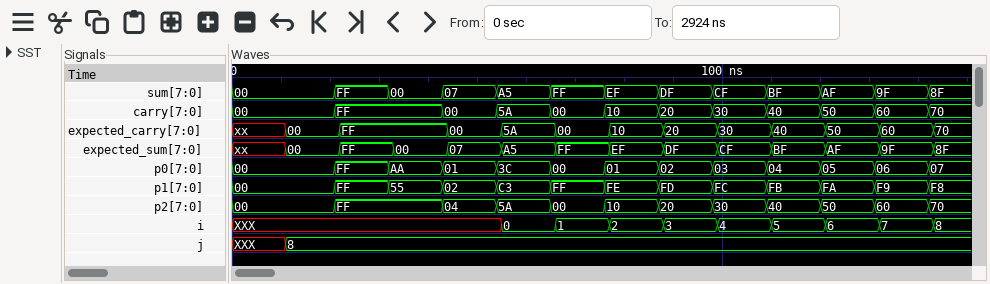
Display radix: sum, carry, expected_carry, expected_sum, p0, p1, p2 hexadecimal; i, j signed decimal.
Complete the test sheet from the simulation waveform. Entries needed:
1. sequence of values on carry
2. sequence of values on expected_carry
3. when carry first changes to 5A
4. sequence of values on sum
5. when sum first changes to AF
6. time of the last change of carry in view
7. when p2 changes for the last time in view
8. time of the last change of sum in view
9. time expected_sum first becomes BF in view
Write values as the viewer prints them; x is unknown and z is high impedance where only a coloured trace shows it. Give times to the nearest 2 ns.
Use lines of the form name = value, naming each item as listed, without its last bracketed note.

sequence of values on carry = 00, FF, 00, 5A, 00, 10, 20, 30, 40, 50, 60, 70
sequence of values on expected_carry = xx, 00, FF, 00, 5A, 00, 10, 20, 30, 40, 50, 60, 70
when carry first changes to 5A = 54 ns
sequence of values on sum = 00, FF, 00, 07, A5, FF, EF, DF, CF, BF, AF, 9F, 8F
when sum first changes to AF = 120 ns
time of the last change of carry in view = 142 ns
when p2 changes for the last time in view = 142 ns
time of the last change of sum in view = 142 ns
time expected_sum first becomes BF in view = 110 ns
